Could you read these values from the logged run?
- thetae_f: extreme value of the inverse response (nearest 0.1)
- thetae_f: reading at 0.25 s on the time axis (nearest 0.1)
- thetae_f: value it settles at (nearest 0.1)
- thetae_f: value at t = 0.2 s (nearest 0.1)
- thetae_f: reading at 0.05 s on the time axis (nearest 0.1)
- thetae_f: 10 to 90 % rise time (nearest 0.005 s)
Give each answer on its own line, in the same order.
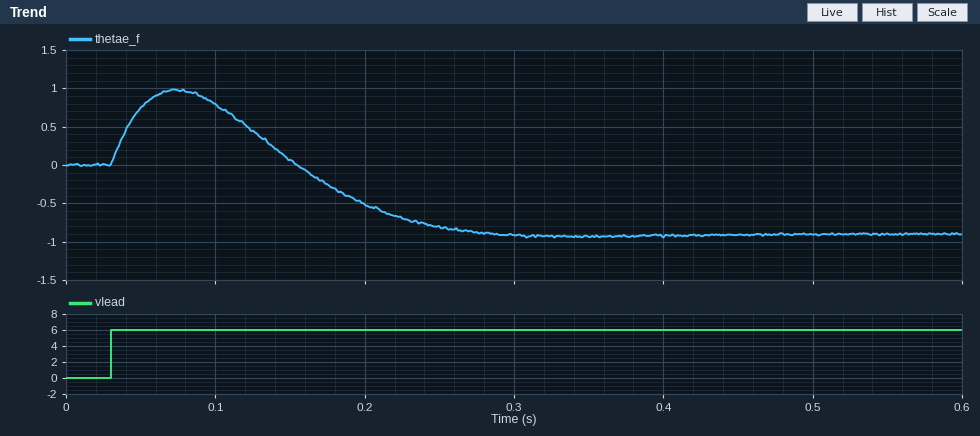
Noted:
1.0
-0.8
-0.9
-0.5
0.7
0.090 s
